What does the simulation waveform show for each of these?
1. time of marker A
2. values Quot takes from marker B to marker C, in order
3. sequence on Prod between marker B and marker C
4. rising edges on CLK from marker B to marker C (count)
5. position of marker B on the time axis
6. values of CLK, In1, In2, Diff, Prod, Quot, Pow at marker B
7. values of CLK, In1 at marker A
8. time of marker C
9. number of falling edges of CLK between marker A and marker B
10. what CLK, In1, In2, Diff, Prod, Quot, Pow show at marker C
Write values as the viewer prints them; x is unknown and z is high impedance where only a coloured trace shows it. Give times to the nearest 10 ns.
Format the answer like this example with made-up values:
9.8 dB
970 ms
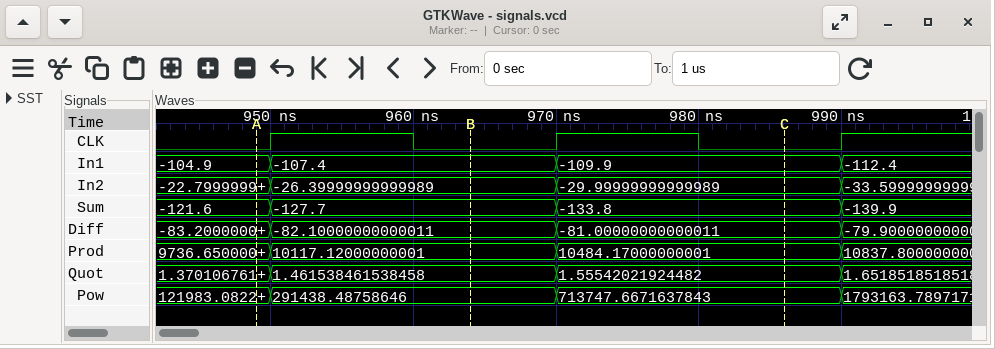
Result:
950 ns
1.461538461538458, 1.55542021924482
10117.12000000001, 10484.17000000001
1
960 ns
CLK=0, In1=-107.4, In2=-26.39999999999989, Diff=-82.10000000000011, Prod=10117.12000000001, Quot=1.461538461538458, Pow=291438.48758646
CLK=0, In1=-104.9
990 ns
1
CLK=0, In1=-109.9, In2=-29.99999999999989, Diff=-81.00000000000011, Prod=10484.17000000001, Quot=1.55542021924482, Pow=713747.6671637843
